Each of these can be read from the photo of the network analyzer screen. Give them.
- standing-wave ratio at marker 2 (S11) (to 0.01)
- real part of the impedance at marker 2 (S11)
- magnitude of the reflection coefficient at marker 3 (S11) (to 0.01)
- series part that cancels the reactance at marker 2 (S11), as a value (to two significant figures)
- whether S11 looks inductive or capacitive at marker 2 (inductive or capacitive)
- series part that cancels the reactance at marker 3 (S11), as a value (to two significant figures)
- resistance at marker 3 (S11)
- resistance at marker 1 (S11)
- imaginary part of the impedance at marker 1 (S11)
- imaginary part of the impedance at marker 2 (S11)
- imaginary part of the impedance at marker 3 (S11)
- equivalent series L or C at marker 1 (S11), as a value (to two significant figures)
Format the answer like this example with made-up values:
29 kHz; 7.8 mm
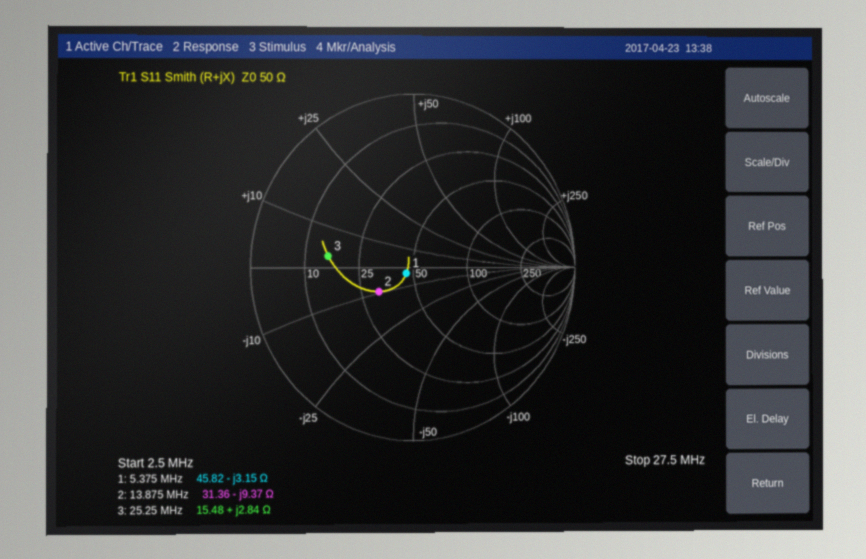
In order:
1.68; 31.36 Ω; 0.53; 110 nH; capacitive; 2.2 nF; 15.48 Ω; 45.82 Ω; -3.15 Ω; -9.37 Ω; +2.84 Ω; 9.4 nF
